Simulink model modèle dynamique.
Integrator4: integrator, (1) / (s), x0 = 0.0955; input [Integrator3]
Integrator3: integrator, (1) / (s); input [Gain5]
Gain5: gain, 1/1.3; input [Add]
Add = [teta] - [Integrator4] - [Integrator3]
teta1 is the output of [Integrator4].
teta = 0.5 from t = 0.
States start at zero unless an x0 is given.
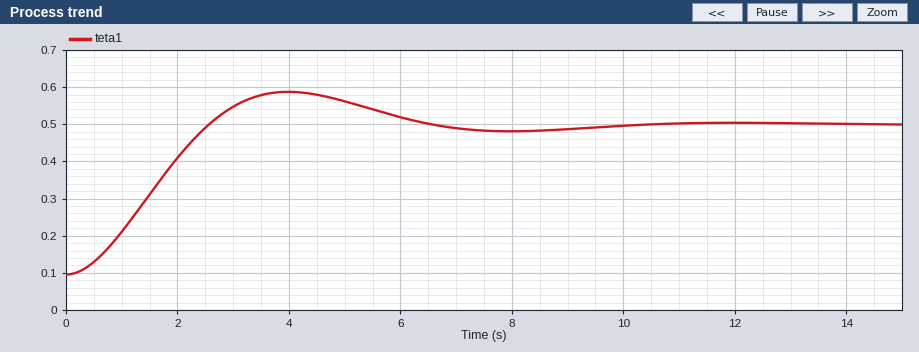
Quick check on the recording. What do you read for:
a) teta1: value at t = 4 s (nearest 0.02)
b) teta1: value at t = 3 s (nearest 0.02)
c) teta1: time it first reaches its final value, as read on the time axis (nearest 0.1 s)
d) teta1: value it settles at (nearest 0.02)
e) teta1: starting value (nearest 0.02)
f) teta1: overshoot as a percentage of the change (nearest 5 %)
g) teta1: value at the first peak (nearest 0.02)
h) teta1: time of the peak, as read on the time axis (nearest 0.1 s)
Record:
0.58
0.54
2.6 s
0.50
0.10
20 %
0.58
4.0 s
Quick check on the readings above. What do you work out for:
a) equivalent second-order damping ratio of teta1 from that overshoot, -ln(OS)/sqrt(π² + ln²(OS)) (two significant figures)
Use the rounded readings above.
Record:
0.46
